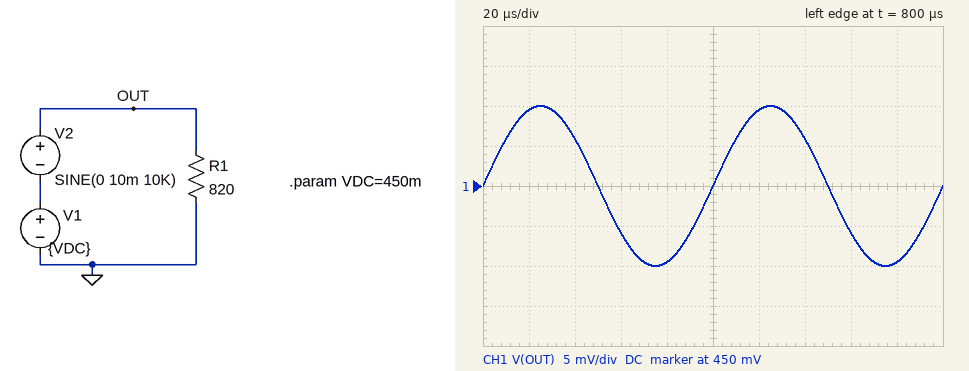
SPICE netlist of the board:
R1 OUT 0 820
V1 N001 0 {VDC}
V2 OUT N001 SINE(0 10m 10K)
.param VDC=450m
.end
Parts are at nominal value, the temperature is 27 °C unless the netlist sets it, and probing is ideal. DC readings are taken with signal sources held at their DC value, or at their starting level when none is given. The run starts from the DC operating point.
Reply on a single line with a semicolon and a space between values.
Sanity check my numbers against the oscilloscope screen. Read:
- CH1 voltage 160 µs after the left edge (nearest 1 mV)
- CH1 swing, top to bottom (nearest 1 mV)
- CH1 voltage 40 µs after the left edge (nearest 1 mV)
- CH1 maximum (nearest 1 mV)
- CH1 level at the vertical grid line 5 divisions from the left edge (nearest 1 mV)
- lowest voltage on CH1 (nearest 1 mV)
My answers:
444 mV; 20 mV; 456 mV; 460 mV; 450 mV; 440 mV
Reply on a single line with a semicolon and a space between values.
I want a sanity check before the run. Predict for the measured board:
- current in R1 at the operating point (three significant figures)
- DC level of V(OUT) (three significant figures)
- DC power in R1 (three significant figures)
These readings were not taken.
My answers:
549 µA; 450 mV; 247 µW
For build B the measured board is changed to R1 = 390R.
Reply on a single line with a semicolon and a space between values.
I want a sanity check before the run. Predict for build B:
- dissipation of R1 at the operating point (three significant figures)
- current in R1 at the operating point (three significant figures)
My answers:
519 µW; 1.15 mA
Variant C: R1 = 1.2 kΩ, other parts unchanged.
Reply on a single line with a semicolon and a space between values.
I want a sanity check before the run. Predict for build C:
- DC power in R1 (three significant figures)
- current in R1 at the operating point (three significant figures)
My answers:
169 µW; 375 µA
